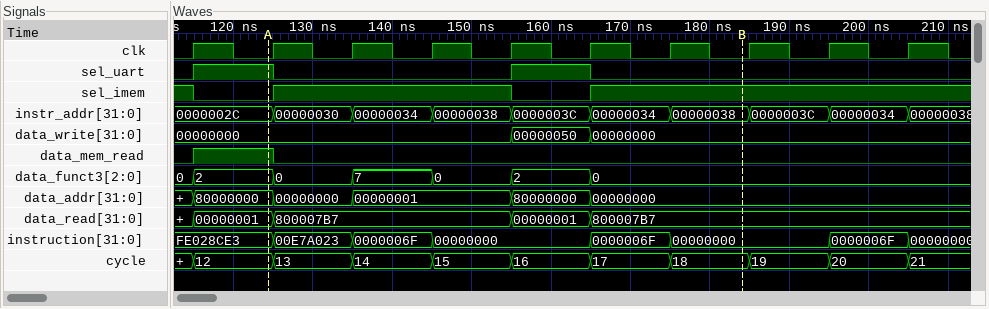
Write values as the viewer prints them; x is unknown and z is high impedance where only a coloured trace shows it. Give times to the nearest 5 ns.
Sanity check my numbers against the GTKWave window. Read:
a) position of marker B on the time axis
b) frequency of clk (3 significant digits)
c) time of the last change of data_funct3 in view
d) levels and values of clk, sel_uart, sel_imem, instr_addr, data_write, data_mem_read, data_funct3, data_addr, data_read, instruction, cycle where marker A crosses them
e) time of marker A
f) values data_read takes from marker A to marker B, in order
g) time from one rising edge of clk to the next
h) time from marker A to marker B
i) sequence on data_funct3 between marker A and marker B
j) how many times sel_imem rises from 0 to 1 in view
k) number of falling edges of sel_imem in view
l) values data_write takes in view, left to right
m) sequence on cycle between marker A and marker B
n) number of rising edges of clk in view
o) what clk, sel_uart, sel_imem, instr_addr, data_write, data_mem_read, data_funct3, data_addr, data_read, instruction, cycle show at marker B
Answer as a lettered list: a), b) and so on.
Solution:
a) 185 ns
b) 100 MHz
c) 165 ns
d) clk=0, sel_uart=1, sel_imem=0, instr_addr=0000002C, data_write=00000000, data_mem_read=1, data_funct3=2, data_addr=80000000, data_read=00000001, instruction=FE028CE3, cycle=12
e) 125 ns
f) 00000001, 800007B7, 00000001, 800007B7
g) 10 ns
h) 60 ns
i) 2, 0, 7, 0, 2, 0
j) 2
k) 2
l) 00000000, 00000050, 00000000
m) 12, 13, 14, 15, 16, 17, 18
n) 10
o) clk=0, sel_uart=0, sel_imem=1, instr_addr=00000038, data_write=00000000, data_mem_read=0, data_funct3=0, data_addr=00000000, data_read=800007B7, instruction=00000000, cycle=18
